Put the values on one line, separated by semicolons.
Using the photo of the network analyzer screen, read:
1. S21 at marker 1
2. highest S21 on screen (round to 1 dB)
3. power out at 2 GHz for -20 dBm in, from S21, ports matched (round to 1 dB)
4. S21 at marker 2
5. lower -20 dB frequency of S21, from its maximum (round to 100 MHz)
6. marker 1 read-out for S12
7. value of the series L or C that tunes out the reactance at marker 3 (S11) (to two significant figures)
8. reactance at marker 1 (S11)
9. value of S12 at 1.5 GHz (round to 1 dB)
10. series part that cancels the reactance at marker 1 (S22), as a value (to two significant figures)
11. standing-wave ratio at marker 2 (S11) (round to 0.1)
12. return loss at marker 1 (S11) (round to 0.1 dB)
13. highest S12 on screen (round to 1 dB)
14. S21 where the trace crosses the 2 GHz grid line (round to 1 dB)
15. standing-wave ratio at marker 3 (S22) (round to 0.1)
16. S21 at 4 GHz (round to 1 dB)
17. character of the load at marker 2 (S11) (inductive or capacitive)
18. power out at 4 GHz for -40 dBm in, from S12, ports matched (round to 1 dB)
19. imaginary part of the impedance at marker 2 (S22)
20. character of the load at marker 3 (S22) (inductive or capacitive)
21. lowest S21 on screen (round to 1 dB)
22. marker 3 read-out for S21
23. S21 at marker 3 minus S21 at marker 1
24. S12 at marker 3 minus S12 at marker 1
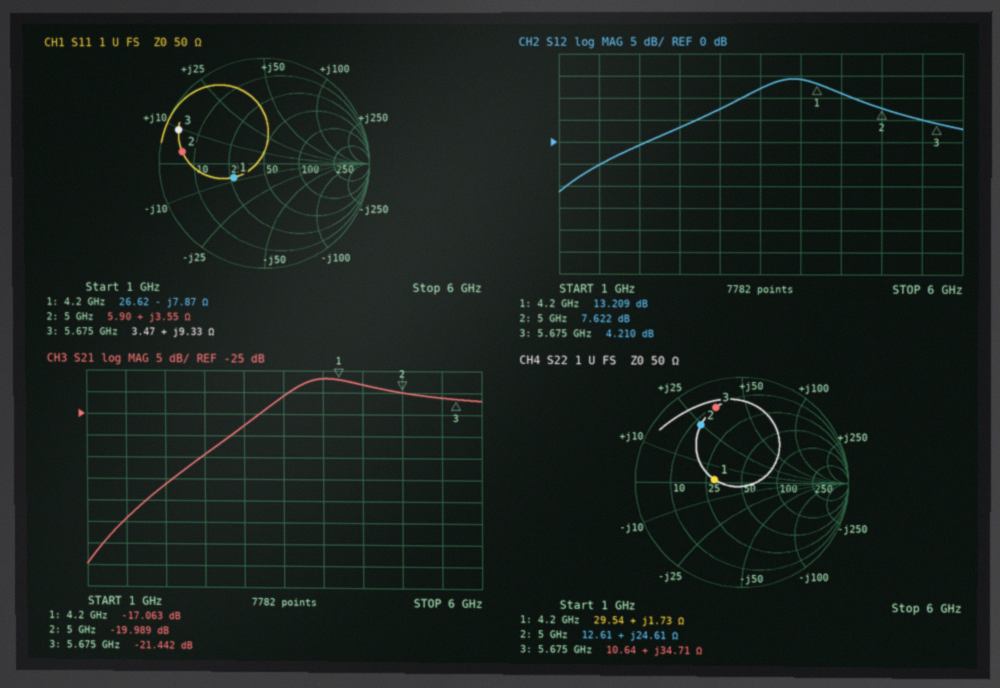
-17.063 dB; -17 dB; -61 dBm; -19.989 dB; 2.3 GHz; 13.209 dB; 3.0 pF; -7.87 Ω; -5 dB; 22 pF; 8.5; 9.9 dB; 14 dB; -41 dB; 7.0; -17 dB; inductive; -26 dBm; +24.61 Ω; inductive; -60 dB; -21.442 dB; -4.379 dB; -8.999 dB
